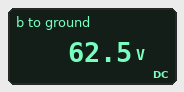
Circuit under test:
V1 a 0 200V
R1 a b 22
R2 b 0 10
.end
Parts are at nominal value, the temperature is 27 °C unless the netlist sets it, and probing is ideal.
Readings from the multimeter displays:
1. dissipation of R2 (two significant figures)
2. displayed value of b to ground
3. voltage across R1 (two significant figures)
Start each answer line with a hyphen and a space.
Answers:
- 390 W
- 62.5 V
- 140 V
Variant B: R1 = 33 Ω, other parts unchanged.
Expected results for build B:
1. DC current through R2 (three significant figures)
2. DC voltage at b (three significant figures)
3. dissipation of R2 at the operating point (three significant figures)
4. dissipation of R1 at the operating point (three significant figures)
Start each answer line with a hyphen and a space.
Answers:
- 4.65 A
- 46.5 V
- 216 W
- 714 W
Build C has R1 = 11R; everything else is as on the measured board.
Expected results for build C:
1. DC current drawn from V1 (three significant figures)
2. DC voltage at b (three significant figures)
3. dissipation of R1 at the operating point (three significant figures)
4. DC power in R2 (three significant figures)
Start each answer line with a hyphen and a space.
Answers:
- 9.52 A
- 95.2 V
- 998 W
- 907 W
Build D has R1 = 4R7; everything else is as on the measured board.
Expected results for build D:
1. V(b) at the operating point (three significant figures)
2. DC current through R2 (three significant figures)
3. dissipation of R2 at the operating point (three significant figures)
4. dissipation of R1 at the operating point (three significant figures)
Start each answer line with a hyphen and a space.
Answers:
- 136 V
- 13.6 A
- 1.85 kW
- 870 W
